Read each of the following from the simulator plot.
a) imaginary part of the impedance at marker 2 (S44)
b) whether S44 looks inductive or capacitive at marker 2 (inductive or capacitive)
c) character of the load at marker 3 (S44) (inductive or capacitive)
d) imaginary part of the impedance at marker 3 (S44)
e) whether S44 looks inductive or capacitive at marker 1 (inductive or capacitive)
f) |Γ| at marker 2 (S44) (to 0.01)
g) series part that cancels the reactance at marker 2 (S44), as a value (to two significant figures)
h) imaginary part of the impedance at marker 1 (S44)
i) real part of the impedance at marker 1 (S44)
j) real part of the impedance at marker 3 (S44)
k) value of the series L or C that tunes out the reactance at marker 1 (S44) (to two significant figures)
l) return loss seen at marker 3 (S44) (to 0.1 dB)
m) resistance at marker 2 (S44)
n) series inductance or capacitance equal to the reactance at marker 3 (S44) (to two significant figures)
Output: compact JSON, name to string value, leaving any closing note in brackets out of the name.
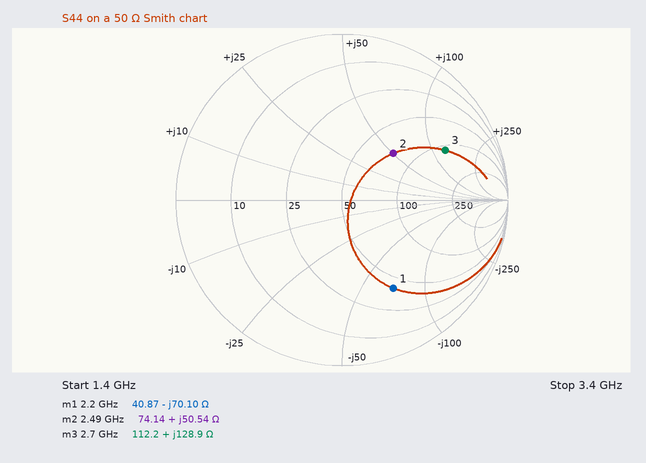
{"imaginary part of the impedance at marker 2": "+50.54 Ω", "whether S44 looks inductive or capacitive at marker 2": "inductive", "character of the load at marker 3 (S44)": "inductive", "imaginary part of the impedance at marker 3": "+128.9 Ω", "whether S44 looks inductive or capacitive at marker 1": "capacitive", "|Γ| at marker 2 (S44)": "0.42", "series part that cancels the reactance at marker 2 (S44), as a value": "1.3 pF", "imaginary part of the impedance at marker 1": "-70.10 Ω", "real part of the impedance at marker 1": "40.87 Ω", "real part of the impedance at marker 3": "112.2 Ω", "value of the series L or C that tunes out the reactance at marker 1 (S44)": "5.1 nH", "return loss seen at marker 3 (S44)": "3.2 dB", "resistance at marker 2": "74.14 Ω", "series inductance or capacitance equal to the reactance at marker 3 (S44)": "7.6 nH"}
